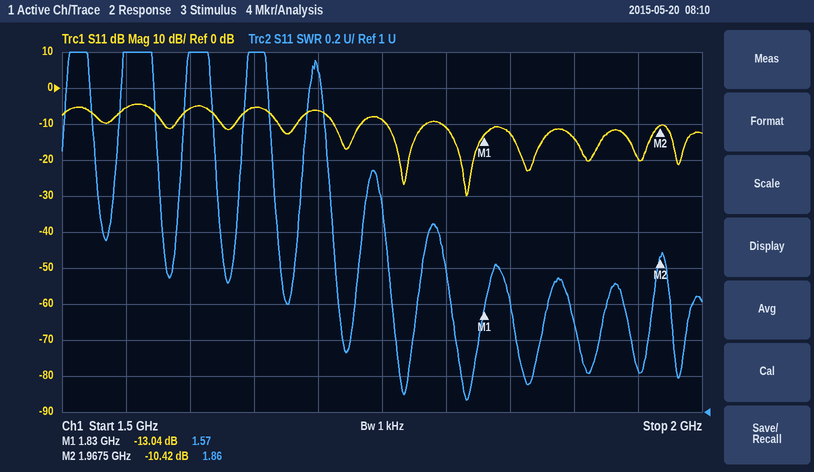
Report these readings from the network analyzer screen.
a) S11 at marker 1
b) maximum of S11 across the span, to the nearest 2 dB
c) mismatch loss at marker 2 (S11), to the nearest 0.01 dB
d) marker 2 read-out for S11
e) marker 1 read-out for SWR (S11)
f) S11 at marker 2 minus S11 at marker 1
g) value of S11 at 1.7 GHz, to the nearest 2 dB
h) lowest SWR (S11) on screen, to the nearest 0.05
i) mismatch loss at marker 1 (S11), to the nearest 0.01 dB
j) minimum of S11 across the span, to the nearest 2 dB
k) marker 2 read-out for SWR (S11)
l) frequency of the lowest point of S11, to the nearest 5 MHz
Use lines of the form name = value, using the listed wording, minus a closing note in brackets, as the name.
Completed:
S11 at marker 1 = -13.04 dB
maximum of S11 across the span, to the nearest 2 dB = -4 dB
mismatch loss at marker 2 (S11), to the nearest 0.01 dB = 0.41 dB
marker 2 read-out for S11 = -10.42 dB
marker 1 read-out for SWR = 1.57
S11 at marker 2 minus S11 at marker 1 = 2.62 dB
value of S11 at 1.7 GHz, to the nearest 2 dB = -6 dB
lowest SWR (S11) on screen, to the nearest 0.05 = 1.05
mismatch loss at marker 1 (S11), to the nearest 0.01 dB = 0.22 dB
minimum of S11 across the span, to the nearest 2 dB = -30 dB
marker 2 read-out for SWR = 1.86
frequency of the lowest point of S11, to the nearest 5 MHz = 1.815 GHz
